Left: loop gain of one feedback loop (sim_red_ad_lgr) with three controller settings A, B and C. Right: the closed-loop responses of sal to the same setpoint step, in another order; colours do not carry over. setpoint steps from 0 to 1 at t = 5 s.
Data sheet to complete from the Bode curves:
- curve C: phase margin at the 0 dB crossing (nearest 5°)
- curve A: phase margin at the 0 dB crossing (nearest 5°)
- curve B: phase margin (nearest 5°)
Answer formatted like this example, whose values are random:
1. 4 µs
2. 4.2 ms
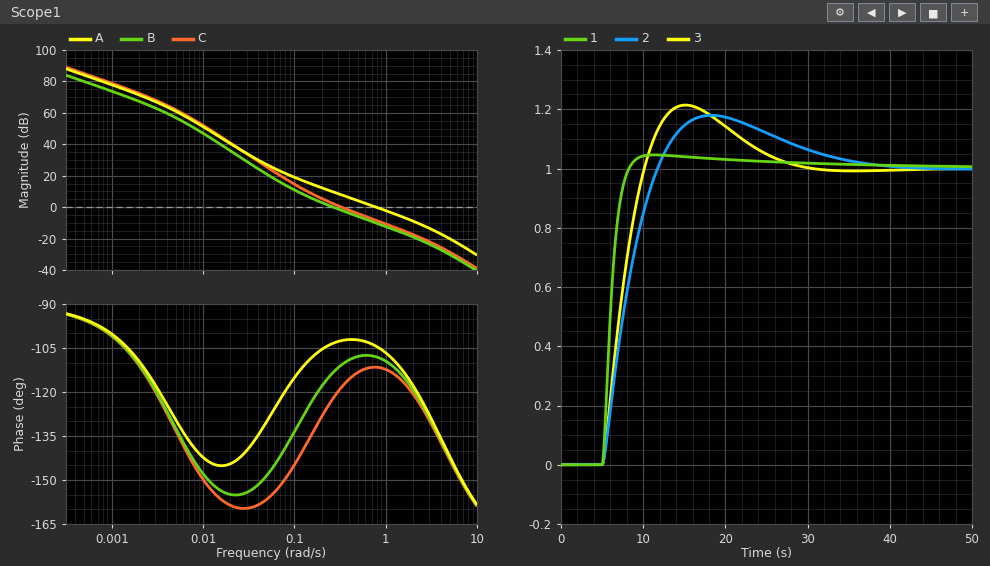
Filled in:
1. 60°
2. 75°
3. 65°
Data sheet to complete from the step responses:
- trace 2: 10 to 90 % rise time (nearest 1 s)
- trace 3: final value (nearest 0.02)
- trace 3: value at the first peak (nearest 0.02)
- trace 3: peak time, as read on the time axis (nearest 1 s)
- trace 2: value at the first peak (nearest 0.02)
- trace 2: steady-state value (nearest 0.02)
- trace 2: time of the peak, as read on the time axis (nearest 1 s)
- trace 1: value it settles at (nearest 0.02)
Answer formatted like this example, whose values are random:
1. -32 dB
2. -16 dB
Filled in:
1. 5 s
2. 1.00
3. 1.22
4. 15 s
5. 1.18
6. 1.00
7. 18 s
8. 1.00
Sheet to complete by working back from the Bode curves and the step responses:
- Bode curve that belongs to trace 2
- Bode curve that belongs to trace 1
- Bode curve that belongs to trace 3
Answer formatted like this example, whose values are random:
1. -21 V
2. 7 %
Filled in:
1. B
2. A
3. C
